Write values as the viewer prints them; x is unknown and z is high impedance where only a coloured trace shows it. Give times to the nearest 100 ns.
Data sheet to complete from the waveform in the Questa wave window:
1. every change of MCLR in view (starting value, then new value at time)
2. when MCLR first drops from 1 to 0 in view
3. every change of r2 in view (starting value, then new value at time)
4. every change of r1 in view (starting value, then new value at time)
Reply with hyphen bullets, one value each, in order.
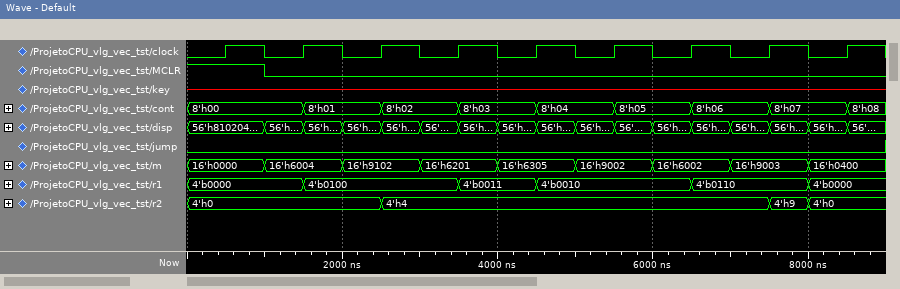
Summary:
- 1, 0 at 1000 ns
- 1000 ns
- 4'h0, 4'h4 at 2500 ns, 4'h9 at 7500 ns, 4'h0 at 8000 ns
- 4'b0000, 4'b0100 at 1500 ns, 4'b0011 at 3500 ns, 4'b0010 at 4500 ns, 4'b0110 at 6500 ns, 4'b0000 at 8000 ns
